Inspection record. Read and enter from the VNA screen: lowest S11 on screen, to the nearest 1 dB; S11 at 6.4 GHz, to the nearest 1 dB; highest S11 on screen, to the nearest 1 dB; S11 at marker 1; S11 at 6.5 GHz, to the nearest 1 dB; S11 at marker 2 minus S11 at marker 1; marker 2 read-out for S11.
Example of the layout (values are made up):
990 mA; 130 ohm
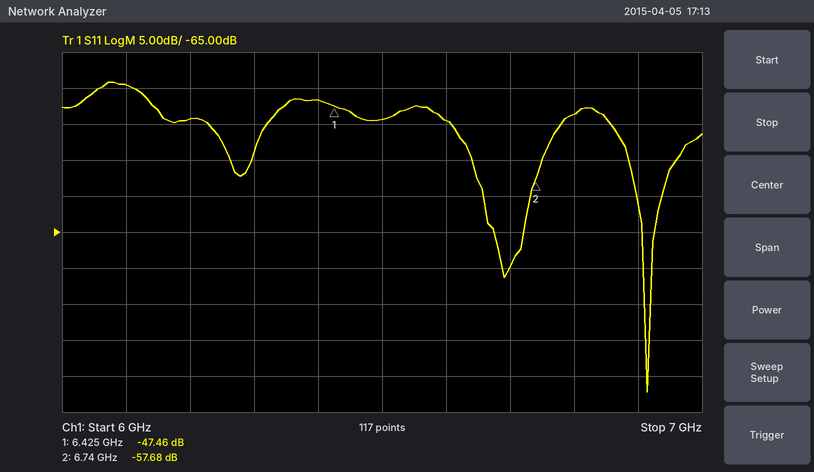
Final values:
-87 dB; -47 dB; -44 dB; -47.46 dB; -49 dB; -10.22 dB; -57.68 dB
